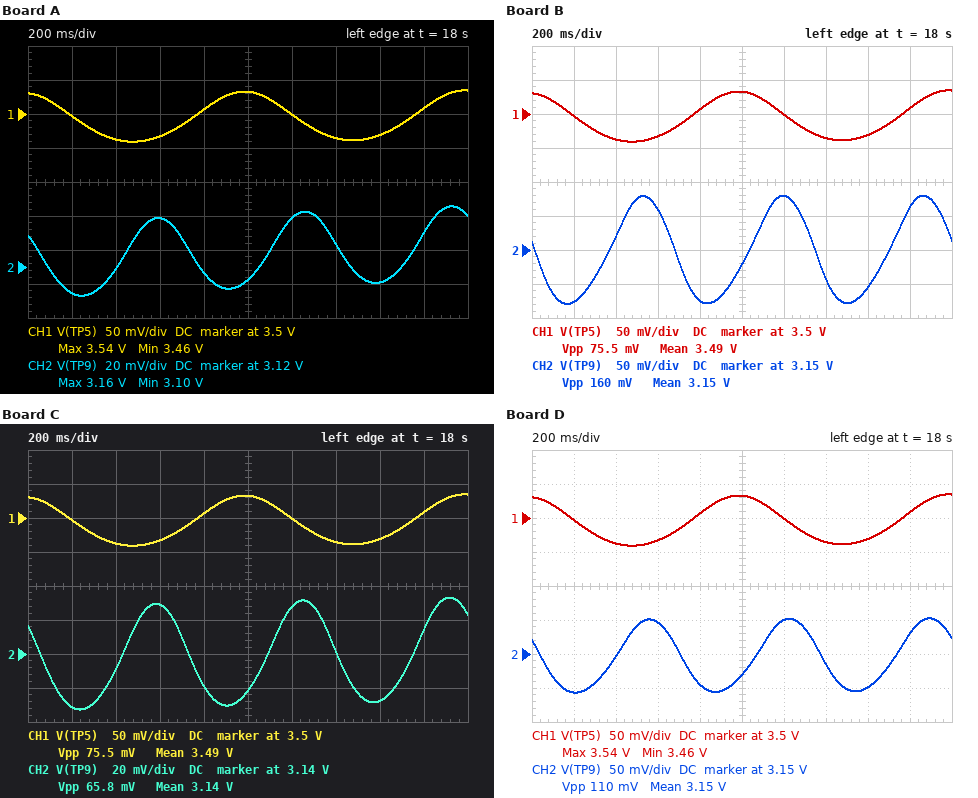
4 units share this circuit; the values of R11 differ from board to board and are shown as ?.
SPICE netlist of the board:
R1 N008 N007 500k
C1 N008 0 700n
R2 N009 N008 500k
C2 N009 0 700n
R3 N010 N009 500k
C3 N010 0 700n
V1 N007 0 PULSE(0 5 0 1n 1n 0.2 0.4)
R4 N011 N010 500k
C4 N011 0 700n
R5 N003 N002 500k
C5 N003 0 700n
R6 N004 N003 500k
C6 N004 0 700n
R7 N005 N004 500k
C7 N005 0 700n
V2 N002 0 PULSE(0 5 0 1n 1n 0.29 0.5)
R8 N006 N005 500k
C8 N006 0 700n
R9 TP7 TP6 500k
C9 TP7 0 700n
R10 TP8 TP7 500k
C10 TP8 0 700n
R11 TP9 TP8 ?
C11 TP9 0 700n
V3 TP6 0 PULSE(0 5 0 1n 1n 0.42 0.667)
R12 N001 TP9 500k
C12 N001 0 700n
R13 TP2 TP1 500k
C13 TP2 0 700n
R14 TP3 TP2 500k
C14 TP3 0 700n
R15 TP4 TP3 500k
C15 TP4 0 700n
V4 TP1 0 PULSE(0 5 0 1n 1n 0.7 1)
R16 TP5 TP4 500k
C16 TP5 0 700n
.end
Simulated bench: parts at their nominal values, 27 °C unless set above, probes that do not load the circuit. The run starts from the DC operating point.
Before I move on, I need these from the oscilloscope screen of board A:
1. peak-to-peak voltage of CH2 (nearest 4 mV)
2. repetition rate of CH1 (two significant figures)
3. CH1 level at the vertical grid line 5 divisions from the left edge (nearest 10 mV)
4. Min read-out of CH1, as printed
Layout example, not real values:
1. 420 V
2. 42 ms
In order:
1. 52 mV
2. 1.0 Hz
3. 3.53 V
4. 3.46 V
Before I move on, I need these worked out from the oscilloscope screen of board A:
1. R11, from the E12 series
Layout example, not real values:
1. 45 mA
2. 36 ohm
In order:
1. 1.2 MΩ
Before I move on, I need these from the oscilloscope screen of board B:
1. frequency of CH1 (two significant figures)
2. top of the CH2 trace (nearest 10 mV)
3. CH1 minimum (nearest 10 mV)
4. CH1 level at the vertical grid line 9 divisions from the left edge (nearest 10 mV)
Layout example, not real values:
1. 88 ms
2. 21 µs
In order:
1. 1.0 Hz
2. 3.23 V
3. 3.46 V
4. 3.51 V
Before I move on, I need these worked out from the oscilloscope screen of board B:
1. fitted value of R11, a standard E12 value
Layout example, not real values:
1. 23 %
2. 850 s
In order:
1. 180 kΩ
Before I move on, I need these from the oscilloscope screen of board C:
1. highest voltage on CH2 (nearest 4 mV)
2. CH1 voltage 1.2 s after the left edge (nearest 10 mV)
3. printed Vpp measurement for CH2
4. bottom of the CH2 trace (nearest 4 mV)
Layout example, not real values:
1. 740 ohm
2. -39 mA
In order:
1. 3.172 V
2. 3.50 V
3. 65.8 mV
4. 3.108 V
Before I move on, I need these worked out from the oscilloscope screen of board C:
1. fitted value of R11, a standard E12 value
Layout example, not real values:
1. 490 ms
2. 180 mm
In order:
1. 820 kΩ
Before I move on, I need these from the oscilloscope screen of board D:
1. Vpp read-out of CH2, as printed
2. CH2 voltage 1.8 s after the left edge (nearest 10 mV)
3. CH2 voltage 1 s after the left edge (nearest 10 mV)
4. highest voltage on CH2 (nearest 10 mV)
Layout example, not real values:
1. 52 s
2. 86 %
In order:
1. 110 mV
2. 3.18 V
3. 3.12 V
4. 3.20 V
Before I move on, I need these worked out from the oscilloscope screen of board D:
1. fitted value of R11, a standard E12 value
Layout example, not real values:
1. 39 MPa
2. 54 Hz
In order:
1. 390 kΩ
